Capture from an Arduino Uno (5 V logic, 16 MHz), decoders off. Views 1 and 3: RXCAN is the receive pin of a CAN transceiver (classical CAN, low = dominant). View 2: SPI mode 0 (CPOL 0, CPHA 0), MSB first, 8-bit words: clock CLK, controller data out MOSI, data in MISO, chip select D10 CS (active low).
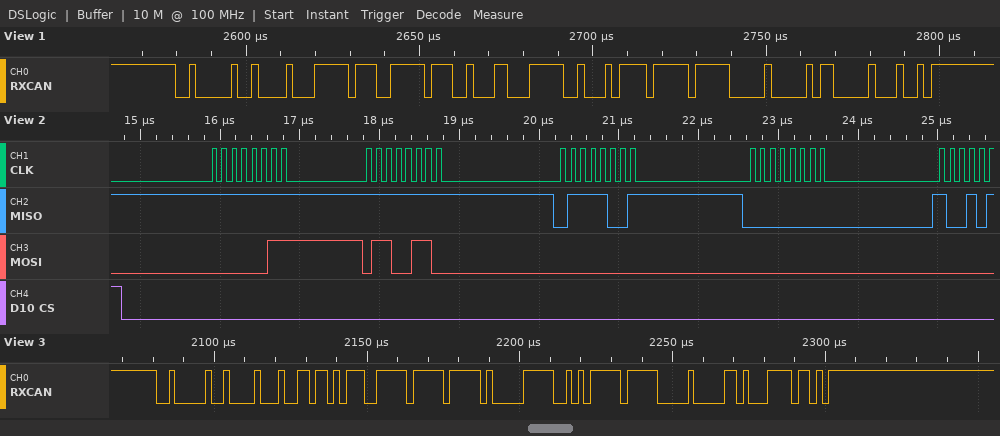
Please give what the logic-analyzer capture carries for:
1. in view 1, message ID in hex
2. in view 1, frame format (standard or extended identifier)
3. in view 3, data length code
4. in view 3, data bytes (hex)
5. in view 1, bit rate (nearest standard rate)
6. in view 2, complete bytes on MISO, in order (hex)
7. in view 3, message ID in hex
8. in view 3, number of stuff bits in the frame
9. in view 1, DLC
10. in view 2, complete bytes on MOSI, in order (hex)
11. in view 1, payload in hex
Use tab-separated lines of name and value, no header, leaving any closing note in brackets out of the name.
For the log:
in view 1, message ID in hex	0x202
in view 1, frame format	standard
in view 3, data length code	8
in view 3, data bytes	9B 5C FF FF 07 AB FF 00
in view 1, bit rate	500 kbit/s
in view 2, complete bytes on MISO, in order	FF FF 79 00
in view 3, message ID in hex	0x202
in view 3, number of stuff bits in the frame	10
in view 1, DLC	8
in view 2, complete bytes on MOSI, in order	03 66 00 00
in view 1, payload in hex	FF 3F C8 C7 D1 7B FF 00
